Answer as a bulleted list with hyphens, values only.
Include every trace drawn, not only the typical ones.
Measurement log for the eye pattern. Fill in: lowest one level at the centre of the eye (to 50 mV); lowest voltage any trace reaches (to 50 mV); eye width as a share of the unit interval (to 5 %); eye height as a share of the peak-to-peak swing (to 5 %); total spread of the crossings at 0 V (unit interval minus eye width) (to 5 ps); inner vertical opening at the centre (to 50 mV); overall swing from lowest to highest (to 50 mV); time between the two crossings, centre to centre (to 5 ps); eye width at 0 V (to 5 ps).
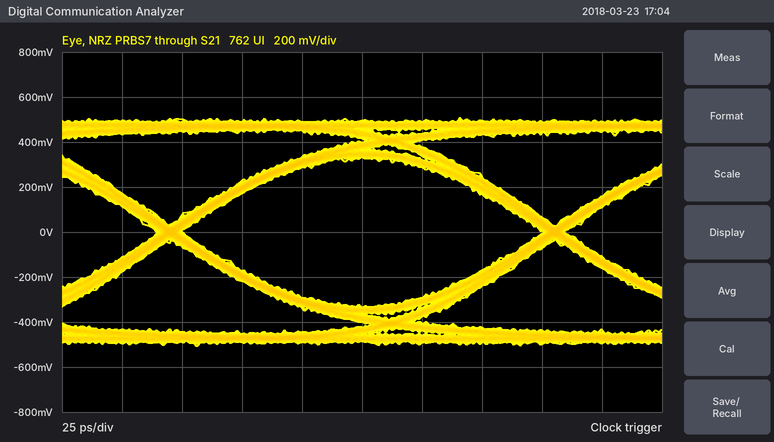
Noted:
- 350 mV
- -500 mV
- 95 %
- 65 %
- 10 ps
- 650 mV
- 1.00 V
- 160 ps
- 150 ps
